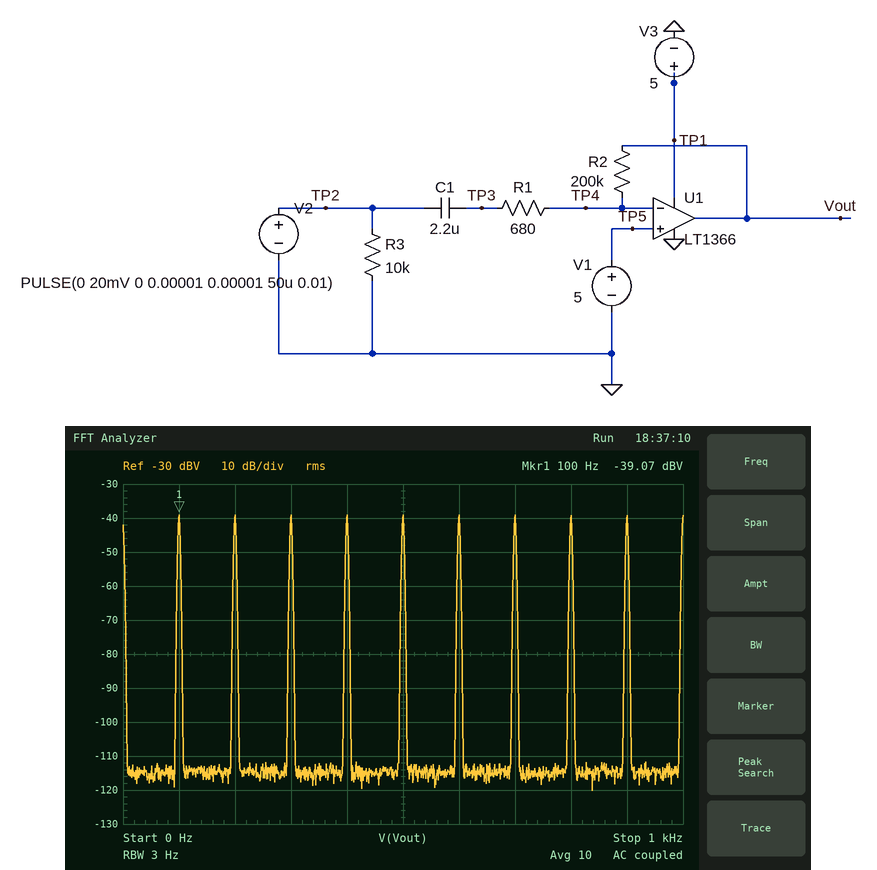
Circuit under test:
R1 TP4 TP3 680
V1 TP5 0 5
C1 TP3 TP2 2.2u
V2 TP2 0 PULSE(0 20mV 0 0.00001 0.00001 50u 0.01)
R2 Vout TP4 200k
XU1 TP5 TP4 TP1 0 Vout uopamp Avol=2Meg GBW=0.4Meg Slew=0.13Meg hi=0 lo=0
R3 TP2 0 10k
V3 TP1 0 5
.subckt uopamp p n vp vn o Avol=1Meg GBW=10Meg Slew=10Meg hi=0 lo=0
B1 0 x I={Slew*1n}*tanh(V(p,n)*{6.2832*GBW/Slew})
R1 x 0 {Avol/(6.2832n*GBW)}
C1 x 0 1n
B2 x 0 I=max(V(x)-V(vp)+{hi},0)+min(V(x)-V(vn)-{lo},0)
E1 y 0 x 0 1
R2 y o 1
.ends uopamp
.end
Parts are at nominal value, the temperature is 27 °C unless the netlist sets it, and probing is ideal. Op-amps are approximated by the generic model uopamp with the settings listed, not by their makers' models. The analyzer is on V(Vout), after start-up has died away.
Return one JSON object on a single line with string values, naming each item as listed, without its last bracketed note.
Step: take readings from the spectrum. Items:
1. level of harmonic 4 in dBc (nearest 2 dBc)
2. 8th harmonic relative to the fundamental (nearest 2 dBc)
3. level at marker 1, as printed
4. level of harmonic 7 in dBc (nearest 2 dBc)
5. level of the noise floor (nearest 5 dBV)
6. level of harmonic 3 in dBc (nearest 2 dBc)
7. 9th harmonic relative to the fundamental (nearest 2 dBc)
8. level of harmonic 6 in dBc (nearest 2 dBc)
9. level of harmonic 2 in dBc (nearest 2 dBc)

{"level of harmonic 4 in dBc": "0 dBc", "8th harmonic relative to the fundamental": "0 dBc", "level at marker 1, as printed": "-39.07 dBV", "level of harmonic 7 in dBc": "0 dBc", "level of the noise floor": "-115 dBV", "level of harmonic 3 in dBc": "0 dBc", "9th harmonic relative to the fundamental": "0 dBc", "level of harmonic 6 in dBc": "0 dBc", "level of harmonic 2 in dBc": "0 dBc"}
